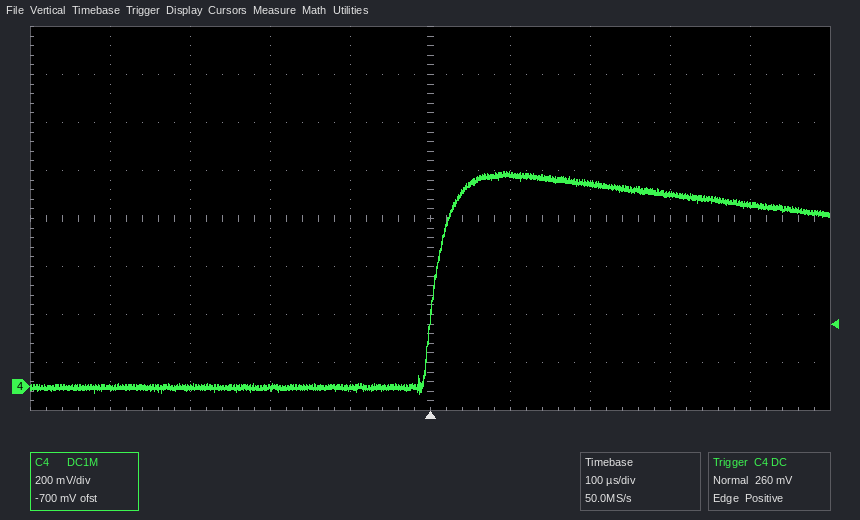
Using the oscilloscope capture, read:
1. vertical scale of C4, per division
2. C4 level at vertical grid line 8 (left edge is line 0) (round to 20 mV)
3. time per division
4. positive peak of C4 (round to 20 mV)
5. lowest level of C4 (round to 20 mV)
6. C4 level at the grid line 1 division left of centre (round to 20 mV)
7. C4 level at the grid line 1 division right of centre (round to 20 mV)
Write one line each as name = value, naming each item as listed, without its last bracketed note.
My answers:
vertical scale of C4, per division = 200 mV
C4 level at vertical grid line 8 (left edge is line 0) = 800 mV
time per division = 100 µs
positive peak of C4 = 900 mV
lowest level of C4 = -40 mV
C4 level at the grid line 1 division left of centre = 0 mV
C4 level at the grid line 1 division right of centre = 880 mV
